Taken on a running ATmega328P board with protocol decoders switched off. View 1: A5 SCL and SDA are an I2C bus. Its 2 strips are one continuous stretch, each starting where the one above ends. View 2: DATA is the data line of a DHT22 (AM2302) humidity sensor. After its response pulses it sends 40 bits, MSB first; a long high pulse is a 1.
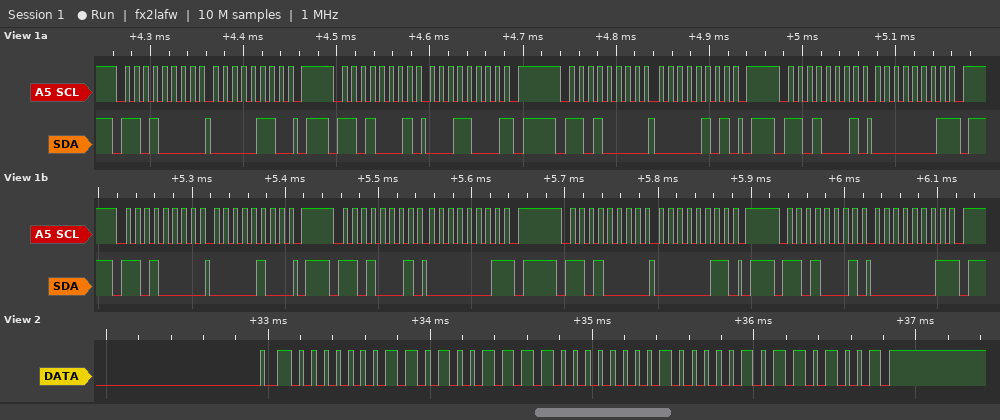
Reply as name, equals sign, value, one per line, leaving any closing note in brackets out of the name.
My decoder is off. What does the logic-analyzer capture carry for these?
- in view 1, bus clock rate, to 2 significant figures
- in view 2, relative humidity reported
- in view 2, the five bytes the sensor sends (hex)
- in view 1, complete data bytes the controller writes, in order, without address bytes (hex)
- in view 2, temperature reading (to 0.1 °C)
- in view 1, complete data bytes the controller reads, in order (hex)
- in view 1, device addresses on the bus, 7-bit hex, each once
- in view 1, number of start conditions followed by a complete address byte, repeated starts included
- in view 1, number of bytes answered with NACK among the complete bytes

in view 1, bus clock rate, to 2 significant figures = 100 kHz
in view 2, relative humidity reported = 42.3 %
in view 2, the five bytes the sensor sends = 01 A7 80 41 69
in view 1, complete data bytes the controller writes, in order, without address bytes = 06 05 04 03
in view 2, temperature reading = -6.5 °C
in view 1, complete data bytes the controller reads, in order = 18 01 01 01
in view 1, device addresses on the bus, 7-bit hex, each once = 0x68
in view 1, number of start conditions followed by a complete address byte, repeated starts included = 8
in view 1, number of bytes answered with NACK among the complete bytes = 4
